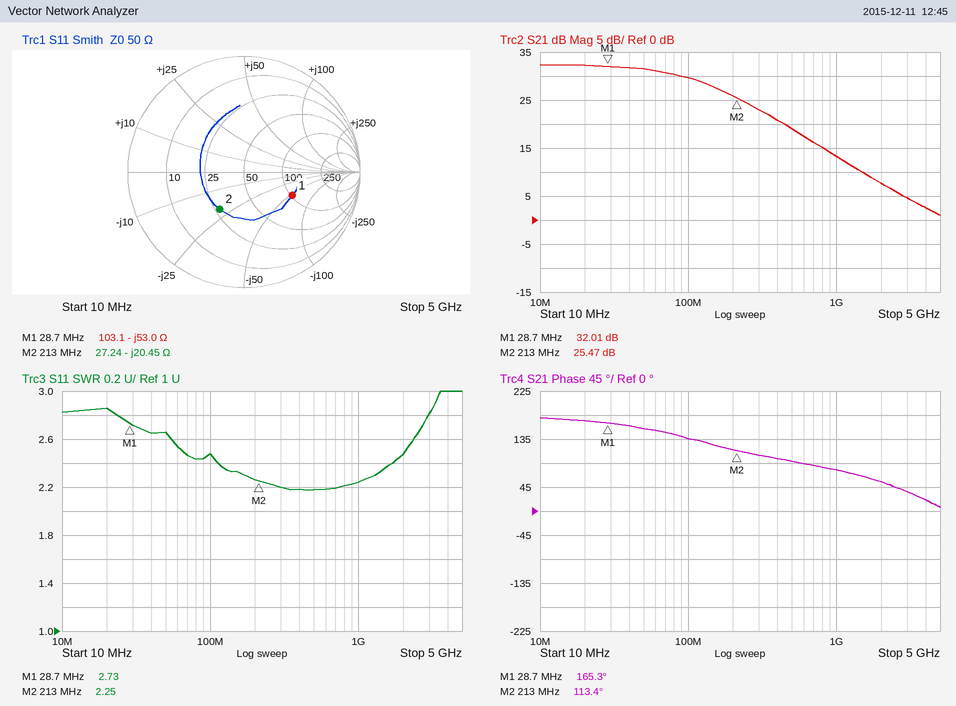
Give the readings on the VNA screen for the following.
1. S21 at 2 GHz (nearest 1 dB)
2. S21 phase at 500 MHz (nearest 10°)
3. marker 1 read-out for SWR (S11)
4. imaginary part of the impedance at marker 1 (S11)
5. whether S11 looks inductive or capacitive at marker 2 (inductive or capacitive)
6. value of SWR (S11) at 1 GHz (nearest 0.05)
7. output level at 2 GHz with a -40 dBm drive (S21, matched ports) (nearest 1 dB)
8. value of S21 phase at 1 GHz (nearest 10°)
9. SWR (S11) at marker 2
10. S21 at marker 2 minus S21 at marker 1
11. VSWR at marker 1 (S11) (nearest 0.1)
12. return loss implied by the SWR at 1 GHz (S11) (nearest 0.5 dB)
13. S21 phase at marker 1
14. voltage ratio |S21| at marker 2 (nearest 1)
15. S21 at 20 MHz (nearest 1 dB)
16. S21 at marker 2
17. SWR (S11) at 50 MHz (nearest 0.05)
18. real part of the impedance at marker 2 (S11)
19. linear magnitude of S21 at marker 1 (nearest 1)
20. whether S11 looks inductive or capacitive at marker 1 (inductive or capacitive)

8 dB
90°
2.73
-53.0 Ω
capacitive
2.25
-32 dBm
80°
2.25
-6.54 dB
2.7
8.5 dB
165.3°
19
32 dB
25.47 dB
2.65
27.24 Ω
40
capacitive
